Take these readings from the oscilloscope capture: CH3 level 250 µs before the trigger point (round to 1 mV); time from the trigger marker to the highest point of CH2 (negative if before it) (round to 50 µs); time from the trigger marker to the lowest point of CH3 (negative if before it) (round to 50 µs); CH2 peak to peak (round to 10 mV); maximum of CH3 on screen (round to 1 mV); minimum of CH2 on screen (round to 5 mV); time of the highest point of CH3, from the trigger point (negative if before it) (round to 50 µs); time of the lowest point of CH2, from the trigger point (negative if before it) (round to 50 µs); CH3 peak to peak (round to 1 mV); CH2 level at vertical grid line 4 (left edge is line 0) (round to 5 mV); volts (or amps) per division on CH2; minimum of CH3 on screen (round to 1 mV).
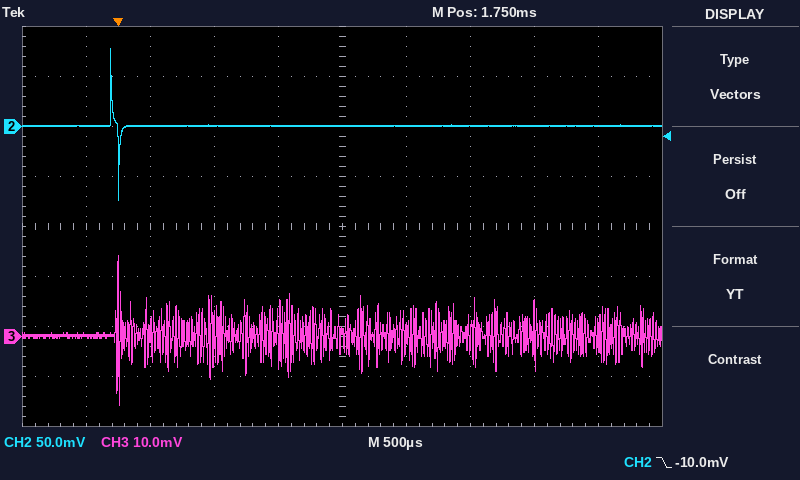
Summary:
0 mV
-50 µs
0 µs
150 mV
16 mV
-75 mV
0 µs
0 µs
30 mV
0 mV
50 mV
-14 mV
